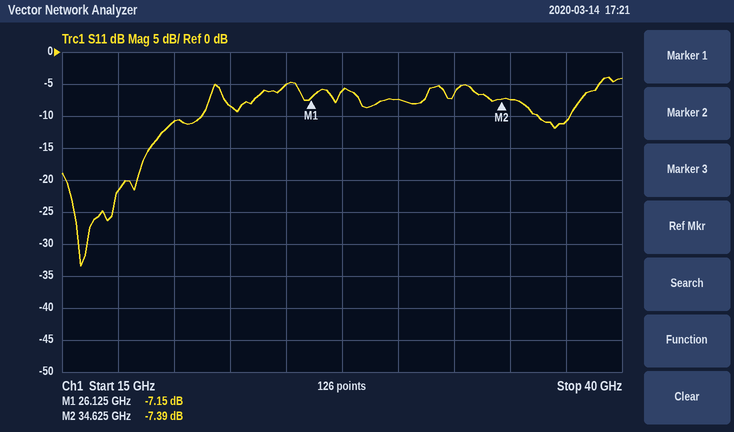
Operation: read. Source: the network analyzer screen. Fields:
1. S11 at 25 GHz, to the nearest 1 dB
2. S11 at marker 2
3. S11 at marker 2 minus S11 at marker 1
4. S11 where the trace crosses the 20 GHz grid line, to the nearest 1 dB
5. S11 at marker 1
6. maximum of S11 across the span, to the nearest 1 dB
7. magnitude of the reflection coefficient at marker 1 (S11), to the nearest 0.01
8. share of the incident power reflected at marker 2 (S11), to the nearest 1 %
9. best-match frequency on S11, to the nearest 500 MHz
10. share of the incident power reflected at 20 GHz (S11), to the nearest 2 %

-5 dB
-7.39 dB
-0.24 dB
-11 dB
-7.15 dB
-4 dB
0.44
18 %
16.0 GHz
8 %
